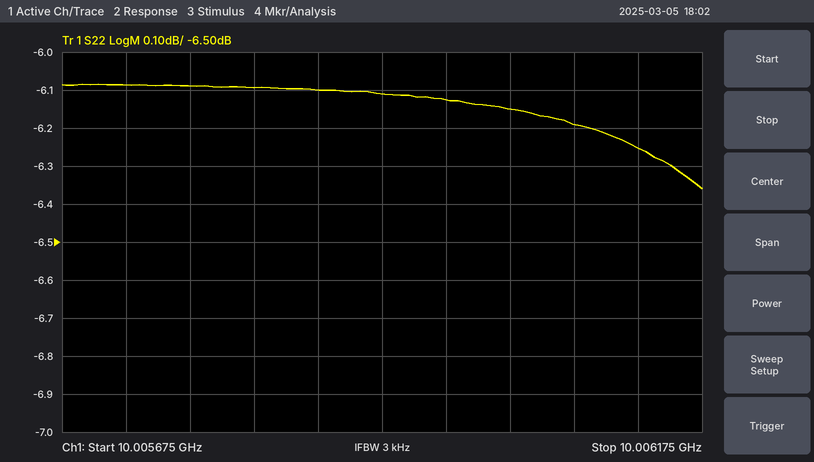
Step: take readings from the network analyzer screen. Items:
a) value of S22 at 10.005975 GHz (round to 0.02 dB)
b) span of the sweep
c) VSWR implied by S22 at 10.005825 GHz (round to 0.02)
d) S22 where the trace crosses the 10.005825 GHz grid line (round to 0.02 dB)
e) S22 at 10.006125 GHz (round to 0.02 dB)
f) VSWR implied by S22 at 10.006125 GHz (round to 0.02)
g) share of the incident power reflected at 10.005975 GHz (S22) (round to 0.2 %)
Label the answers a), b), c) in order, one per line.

a) -6.12 dB
b) 500 kHz
c) 2.96
d) -6.10 dB
e) -6.26 dB
f) 2.90
g) 24.4 %
